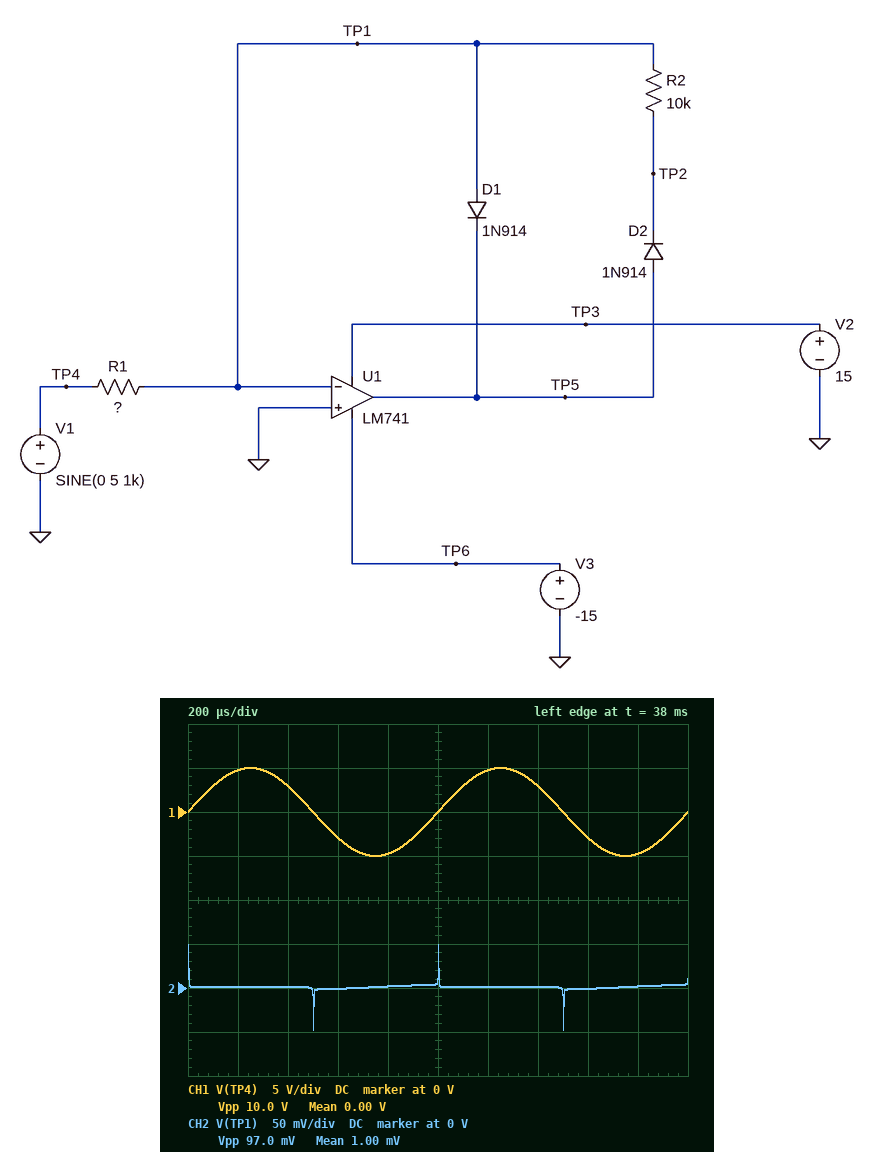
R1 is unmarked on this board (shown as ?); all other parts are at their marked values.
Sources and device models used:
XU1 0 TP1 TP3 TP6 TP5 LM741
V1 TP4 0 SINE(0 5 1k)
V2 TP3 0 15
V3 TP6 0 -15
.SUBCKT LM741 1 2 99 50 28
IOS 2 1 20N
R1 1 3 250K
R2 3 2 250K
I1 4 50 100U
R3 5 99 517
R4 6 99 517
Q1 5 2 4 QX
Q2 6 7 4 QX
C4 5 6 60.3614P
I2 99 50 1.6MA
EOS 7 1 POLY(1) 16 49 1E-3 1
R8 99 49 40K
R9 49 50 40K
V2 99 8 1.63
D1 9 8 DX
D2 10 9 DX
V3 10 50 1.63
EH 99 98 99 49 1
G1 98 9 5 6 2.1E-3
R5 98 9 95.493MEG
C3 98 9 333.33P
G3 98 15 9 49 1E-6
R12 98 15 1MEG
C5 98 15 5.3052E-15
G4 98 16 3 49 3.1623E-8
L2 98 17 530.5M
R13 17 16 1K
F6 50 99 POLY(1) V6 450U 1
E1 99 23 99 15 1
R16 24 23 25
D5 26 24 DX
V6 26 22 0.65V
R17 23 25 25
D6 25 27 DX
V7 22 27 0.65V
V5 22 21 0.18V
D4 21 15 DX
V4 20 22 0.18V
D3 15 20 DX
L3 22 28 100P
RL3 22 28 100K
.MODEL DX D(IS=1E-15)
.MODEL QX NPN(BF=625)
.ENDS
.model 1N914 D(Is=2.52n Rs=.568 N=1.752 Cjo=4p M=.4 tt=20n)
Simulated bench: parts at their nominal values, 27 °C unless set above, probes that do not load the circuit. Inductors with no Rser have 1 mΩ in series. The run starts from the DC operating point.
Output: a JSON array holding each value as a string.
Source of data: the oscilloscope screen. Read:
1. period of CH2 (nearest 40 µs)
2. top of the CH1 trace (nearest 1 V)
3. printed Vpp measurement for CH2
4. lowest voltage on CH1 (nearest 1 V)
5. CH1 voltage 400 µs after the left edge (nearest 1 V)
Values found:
["1.00 ms", "5 V", "97.0 mV", "-5 V", "3 V"]
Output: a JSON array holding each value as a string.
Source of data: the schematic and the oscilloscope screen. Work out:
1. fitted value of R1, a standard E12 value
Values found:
["22 kΩ"]
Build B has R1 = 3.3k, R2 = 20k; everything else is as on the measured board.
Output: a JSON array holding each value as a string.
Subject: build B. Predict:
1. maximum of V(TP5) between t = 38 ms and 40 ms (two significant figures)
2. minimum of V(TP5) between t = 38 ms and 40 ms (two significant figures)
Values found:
["14 V", "-600 mV"]
